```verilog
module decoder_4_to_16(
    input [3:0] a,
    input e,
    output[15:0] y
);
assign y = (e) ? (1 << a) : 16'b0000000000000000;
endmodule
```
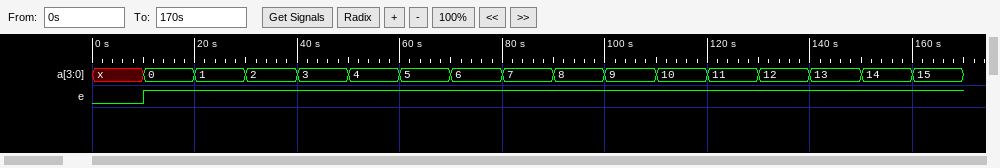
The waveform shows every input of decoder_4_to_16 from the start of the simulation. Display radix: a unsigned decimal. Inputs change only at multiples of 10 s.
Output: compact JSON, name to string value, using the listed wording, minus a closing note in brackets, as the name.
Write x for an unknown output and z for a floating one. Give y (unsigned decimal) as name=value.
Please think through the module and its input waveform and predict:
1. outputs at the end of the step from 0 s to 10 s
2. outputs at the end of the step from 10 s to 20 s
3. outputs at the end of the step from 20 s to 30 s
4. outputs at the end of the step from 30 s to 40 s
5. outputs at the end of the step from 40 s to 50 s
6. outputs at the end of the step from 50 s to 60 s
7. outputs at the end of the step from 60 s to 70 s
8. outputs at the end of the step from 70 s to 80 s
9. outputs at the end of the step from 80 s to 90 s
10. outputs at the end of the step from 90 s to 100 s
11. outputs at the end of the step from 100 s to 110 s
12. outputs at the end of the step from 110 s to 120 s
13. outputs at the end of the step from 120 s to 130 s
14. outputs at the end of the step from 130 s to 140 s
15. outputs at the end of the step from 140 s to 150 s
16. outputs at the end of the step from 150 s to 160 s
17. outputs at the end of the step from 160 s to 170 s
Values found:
{"outputs at the end of the step from 0 s to 10 s": "y=0", "outputs at the end of the step from 10 s to 20 s": "y=1", "outputs at the end of the step from 20 s to 30 s": "y=2", "outputs at the end of the step from 30 s to 40 s": "y=4", "outputs at the end of the step from 40 s to 50 s": "y=8", "outputs at the end of the step from 50 s to 60 s": "y=16", "outputs at the end of the step from 60 s to 70 s": "y=32", "outputs at the end of the step from 70 s to 80 s": "y=64", "outputs at the end of the step from 80 s to 90 s": "y=128", "outputs at the end of the step from 90 s to 100 s": "y=256", "outputs at the end of the step from 100 s to 110 s": "y=512", "outputs at the end of the step from 110 s to 120 s": "y=1024", "outputs at the end of the step from 120 s to 130 s": "y=2048", "outputs at the end of the step from 130 s to 140 s": "y=4096", "outputs at the end of the step from 140 s to 150 s": "y=8192", "outputs at the end of the step from 150 s to 160 s": "y=16384", "outputs at the end of the step from 160 s to 170 s": "y=32768"}
